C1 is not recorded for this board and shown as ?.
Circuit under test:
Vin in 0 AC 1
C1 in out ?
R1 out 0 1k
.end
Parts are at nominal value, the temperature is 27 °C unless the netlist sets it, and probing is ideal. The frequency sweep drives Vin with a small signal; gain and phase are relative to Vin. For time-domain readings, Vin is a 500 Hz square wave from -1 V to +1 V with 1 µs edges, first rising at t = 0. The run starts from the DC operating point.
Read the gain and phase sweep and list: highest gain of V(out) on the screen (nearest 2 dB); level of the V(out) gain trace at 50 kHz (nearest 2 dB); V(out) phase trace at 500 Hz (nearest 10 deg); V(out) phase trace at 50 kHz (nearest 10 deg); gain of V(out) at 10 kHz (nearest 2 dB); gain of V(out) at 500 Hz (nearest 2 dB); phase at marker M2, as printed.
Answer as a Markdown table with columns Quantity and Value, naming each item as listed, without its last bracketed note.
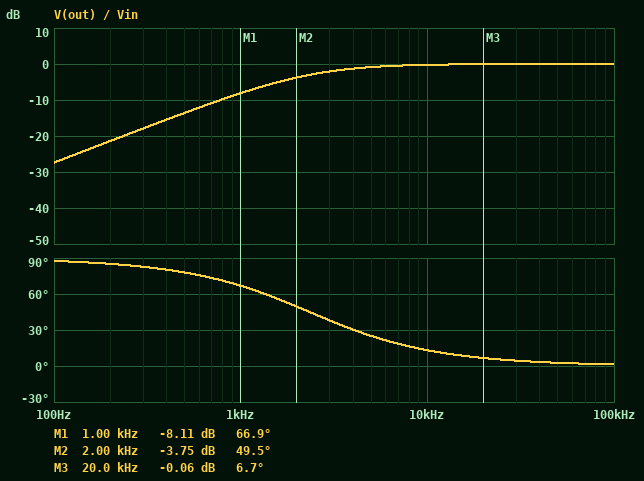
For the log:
| Quantity | Value |
|---|---|
| highest gain of V(out) on the screen | 0 dB |
| level of the V(out) gain trace at 50 kHz | 0 dB |
| V(out) phase trace at 500 Hz | 80 deg |
| V(out) phase trace at 50 kHz | 0 deg |
| gain of V(out) at 10 kHz | 0 dB |
| gain of V(out) at 500 Hz | -14 dB |
| phase at marker M2, as printed | 49.5 deg |
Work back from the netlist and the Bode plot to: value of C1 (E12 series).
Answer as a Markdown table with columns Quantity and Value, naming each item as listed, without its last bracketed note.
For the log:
| Quantity | Value |
|---|---|
| value of C1 | 68 nF |
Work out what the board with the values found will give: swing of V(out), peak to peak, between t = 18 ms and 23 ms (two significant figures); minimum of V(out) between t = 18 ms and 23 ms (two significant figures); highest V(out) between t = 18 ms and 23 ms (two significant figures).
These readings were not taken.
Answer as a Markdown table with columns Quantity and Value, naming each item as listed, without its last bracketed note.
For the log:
| Quantity | Value |
|---|---|
| swing of V(out), peak to peak, between t = 18 ms and 23 ms | 4.0 V |
| minimum of V(out) between t = 18 ms and 23 ms | -2.0 V |
| highest V(out) between t = 18 ms and 23 ms | 2.0 V |
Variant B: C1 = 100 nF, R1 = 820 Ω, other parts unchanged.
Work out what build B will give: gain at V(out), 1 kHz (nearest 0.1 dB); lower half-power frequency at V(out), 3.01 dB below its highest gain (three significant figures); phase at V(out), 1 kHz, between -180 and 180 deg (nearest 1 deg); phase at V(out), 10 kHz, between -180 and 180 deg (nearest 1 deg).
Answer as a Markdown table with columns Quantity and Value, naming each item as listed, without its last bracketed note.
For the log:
| Quantity | Value |
|---|---|
| gain at V(out), 1 kHz | -6.8 dB |
| lower half-power frequency at V(out), 3.01 dB below its highest gain | 1.94 kHz |
| phase at V(out), 1 kHz, between -180 and 180 deg | 63 deg |
| phase at V(out), 10 kHz, between -180 and 180 deg | 11 deg |
